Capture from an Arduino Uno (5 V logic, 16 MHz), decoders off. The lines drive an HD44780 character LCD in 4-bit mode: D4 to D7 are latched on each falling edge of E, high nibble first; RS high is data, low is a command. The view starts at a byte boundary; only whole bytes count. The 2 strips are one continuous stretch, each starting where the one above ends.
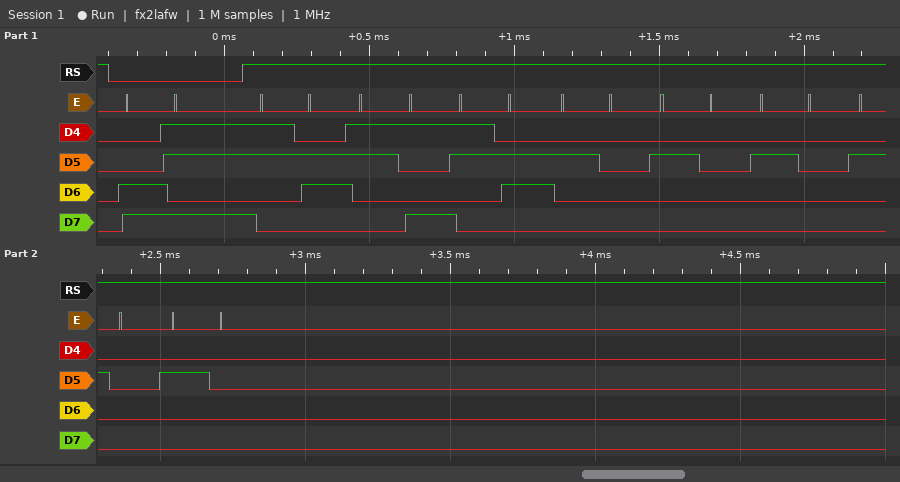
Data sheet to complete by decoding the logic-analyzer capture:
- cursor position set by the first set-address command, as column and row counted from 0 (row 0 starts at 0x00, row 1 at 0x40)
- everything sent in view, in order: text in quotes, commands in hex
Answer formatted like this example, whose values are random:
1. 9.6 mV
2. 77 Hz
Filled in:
1. column 11, row 1
2. 0xCB "696     "
